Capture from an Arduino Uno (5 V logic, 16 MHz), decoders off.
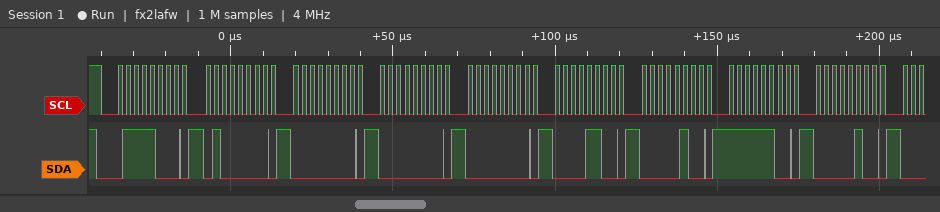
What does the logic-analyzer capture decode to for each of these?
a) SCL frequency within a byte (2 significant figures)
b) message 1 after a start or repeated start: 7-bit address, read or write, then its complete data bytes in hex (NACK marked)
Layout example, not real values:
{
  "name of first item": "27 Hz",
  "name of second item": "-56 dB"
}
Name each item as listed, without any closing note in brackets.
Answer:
{
  "SCL frequency within a byte": "400 kHz",
  "message 1 after a start or repeated start: 7-bit address, read or write, then its complete data bytes in hex": "0x3C write: 40 00 00 00 0C 04 FC 04"
}
